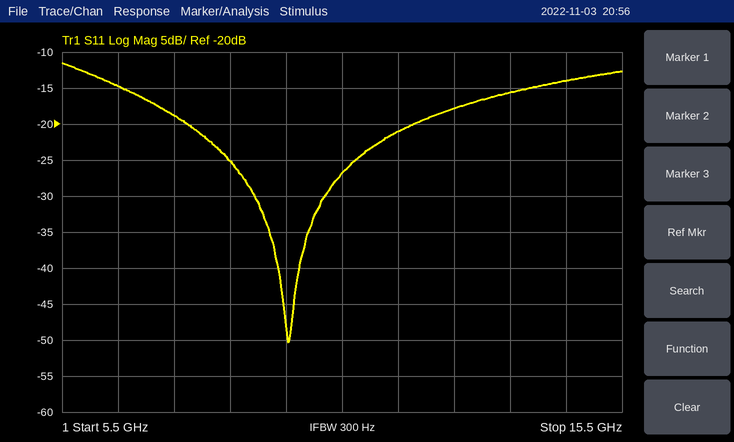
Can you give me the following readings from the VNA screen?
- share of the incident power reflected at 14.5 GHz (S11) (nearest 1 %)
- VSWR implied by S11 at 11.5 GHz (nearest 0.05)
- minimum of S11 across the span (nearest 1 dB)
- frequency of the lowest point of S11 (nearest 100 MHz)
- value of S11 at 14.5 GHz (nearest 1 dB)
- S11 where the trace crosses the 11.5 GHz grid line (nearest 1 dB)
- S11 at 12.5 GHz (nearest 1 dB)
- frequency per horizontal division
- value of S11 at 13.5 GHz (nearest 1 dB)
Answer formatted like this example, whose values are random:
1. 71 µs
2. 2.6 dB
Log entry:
1. 4 %
2. 1.20
3. -50 dB
4. 9.5 GHz
5. -14 dB
6. -21 dB
7. -18 dB
8. 1 GHz
9. -16 dB
